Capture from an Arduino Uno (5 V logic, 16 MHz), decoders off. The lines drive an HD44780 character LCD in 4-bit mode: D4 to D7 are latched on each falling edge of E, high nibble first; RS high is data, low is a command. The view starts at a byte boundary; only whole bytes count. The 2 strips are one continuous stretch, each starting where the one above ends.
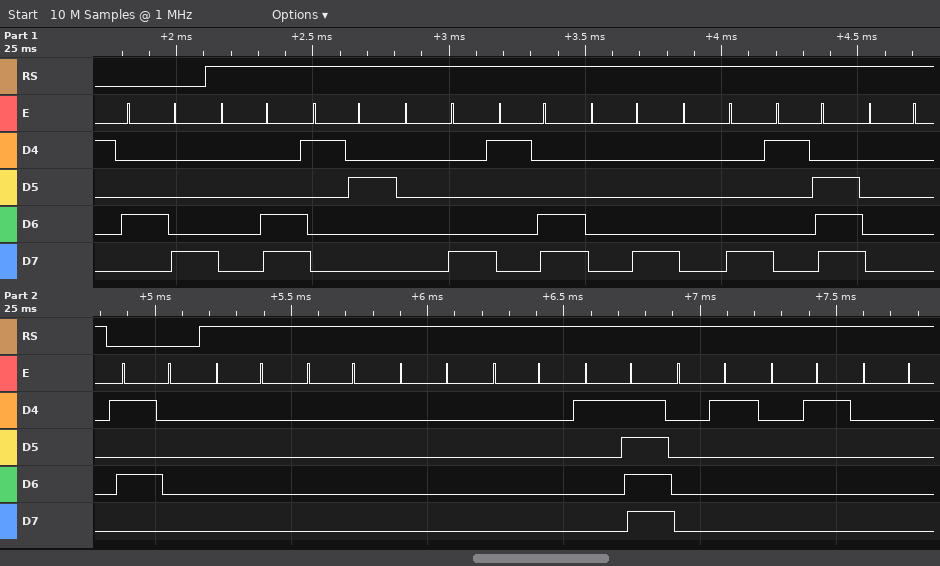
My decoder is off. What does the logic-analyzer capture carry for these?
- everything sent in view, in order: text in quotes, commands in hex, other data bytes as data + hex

0x48 data 0C 12 08 1C 08 08 1E 00 0x50 data 00 00 00 00 1F 01 01 00
